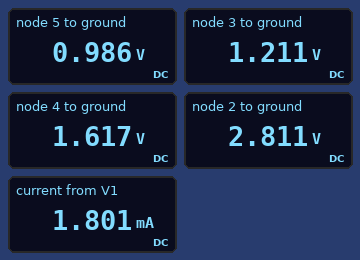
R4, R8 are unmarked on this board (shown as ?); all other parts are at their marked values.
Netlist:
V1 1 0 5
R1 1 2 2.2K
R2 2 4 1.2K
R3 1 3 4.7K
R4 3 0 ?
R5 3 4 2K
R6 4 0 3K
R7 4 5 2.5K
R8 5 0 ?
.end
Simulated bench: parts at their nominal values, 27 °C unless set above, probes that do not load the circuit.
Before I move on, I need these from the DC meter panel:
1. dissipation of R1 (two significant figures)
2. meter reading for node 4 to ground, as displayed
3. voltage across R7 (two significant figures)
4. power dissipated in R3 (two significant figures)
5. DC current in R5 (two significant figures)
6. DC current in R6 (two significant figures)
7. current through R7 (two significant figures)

2.2 mW
1.617 V
630 mV
3.1 mW
200 µA
540 µA
250 µA
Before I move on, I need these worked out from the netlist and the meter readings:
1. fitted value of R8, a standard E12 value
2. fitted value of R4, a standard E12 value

3.9 kΩ
1.2 kΩ
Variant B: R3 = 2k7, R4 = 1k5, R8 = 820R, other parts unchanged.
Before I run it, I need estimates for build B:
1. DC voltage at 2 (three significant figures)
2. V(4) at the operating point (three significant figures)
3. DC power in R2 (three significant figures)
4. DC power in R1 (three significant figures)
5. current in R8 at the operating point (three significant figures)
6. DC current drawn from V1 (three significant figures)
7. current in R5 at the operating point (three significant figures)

2.82 V
1.64 V
1.17 mW
2.15 mW
493 µA
2.20 mA
50.0 µA
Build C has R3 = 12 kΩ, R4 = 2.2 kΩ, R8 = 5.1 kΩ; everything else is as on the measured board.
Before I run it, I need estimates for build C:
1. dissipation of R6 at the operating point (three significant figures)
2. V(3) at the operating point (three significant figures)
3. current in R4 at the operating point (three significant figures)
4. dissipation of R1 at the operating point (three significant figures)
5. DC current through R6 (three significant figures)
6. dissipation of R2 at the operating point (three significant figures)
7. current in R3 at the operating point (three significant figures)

898 µW
1.19 V
542 µA
2.15 mW
547 µA
1.17 mW
317 µA
